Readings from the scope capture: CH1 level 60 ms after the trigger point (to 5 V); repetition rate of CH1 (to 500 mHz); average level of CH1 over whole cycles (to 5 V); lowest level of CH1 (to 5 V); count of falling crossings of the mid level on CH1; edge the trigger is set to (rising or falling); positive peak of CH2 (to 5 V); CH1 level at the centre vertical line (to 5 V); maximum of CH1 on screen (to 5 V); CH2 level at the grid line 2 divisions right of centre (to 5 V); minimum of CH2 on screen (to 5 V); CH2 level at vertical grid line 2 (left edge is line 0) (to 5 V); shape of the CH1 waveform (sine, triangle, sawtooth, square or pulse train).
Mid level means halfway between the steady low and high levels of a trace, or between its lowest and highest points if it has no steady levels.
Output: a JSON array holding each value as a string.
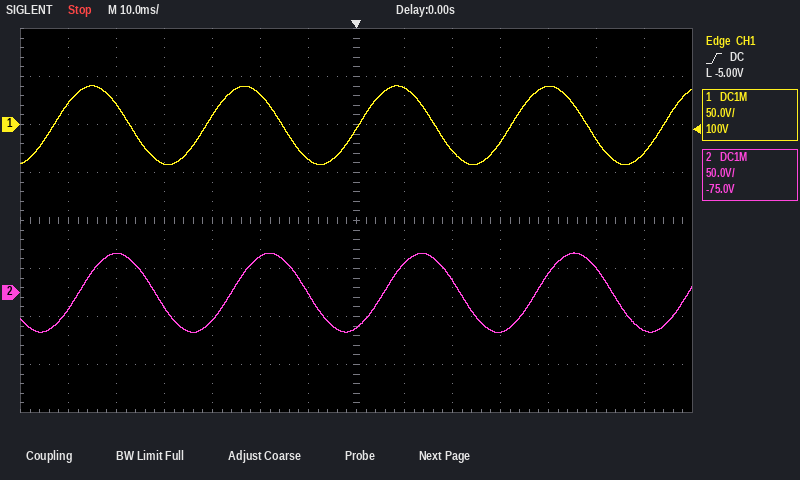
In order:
["-30 V", "31.5 Hz", "0 V", "-40 V", "4", "rising", "40 V", "-5 V", "40 V", "15 V", "-40 V", "40 V", "sine"]
